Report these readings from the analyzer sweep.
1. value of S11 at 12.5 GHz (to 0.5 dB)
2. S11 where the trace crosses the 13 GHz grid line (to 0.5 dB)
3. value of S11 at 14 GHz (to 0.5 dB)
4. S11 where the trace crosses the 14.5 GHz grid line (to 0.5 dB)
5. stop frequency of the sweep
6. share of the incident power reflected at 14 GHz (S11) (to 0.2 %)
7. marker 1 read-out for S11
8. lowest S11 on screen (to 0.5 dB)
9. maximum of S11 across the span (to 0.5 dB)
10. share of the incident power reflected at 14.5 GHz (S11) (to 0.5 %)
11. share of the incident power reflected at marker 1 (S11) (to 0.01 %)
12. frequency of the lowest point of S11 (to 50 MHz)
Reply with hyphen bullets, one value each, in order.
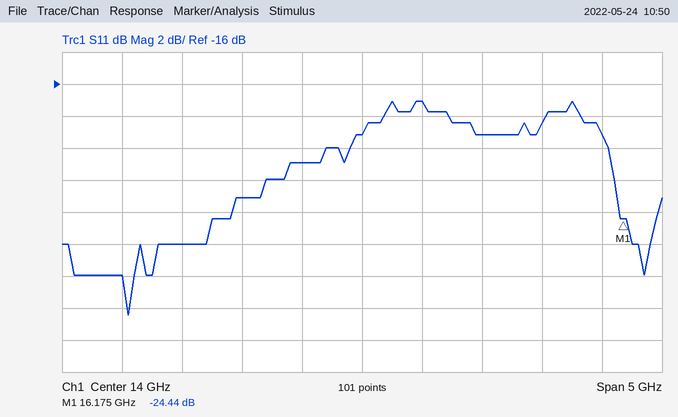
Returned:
- -26.0 dB
- -23.0 dB
- -19.0 dB
- -17.0 dB
- 16.5 GHz
- 1.2 %
- -24.44 dB
- -30.5 dB
- -17.0 dB
- 2.0 %
- 0.36 %
- 12.05 GHz
